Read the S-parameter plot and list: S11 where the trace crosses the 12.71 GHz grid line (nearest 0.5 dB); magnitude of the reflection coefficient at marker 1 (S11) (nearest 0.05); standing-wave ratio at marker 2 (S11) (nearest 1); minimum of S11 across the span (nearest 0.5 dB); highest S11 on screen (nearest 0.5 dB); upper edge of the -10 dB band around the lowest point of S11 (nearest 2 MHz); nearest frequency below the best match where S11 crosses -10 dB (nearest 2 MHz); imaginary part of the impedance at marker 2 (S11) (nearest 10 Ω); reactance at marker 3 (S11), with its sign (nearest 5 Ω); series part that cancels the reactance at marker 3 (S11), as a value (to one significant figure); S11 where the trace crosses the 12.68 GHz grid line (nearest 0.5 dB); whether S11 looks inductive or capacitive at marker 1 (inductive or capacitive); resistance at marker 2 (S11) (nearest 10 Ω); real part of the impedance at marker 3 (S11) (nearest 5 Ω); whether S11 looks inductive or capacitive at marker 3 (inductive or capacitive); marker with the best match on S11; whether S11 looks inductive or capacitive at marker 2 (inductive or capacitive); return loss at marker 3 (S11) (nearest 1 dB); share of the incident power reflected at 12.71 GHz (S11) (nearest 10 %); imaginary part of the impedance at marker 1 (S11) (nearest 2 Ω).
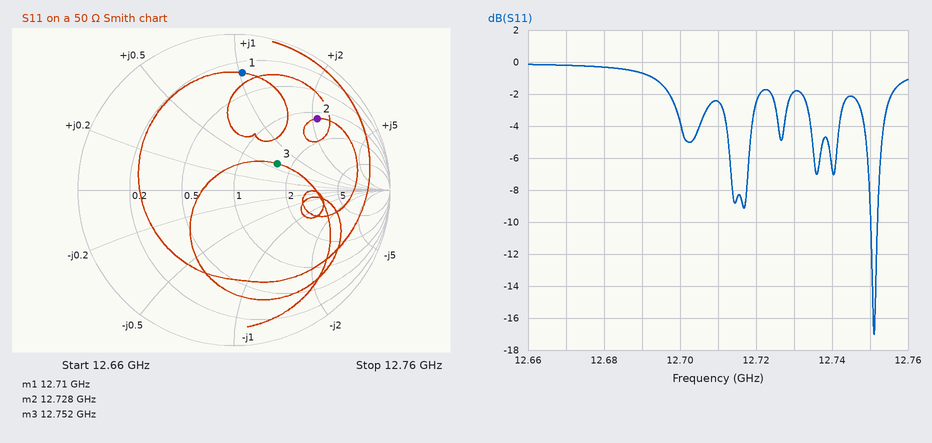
-2.5 dB
0.75
6
-17.0 dB
0.0 dB
12.752 GHz
12.750 GHz
+110 Ω
+30 Ω
400 fF
-0.5 dB
inductive
60 Ω
80 Ω
inductive
marker 3
inductive
10 dB
60 %
+52 Ω
